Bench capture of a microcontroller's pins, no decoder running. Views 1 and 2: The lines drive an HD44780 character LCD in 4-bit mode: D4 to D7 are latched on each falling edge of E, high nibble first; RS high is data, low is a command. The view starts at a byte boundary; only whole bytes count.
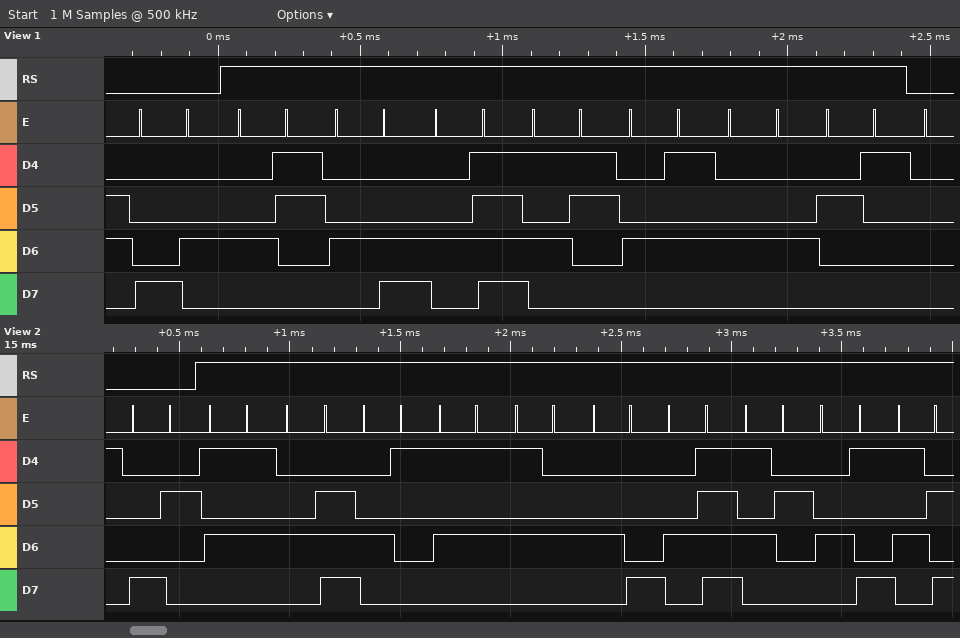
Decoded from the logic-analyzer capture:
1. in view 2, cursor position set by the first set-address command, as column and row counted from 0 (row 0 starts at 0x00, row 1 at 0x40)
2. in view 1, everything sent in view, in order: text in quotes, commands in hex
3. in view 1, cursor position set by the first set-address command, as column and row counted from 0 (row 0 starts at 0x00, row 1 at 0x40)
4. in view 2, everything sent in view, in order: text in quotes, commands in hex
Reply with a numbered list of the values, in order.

1. column 2, row 0
2. 0x84 "CLOSED!"
3. column 4, row 0
4. 0x82 "UNAUTHORIZ"
